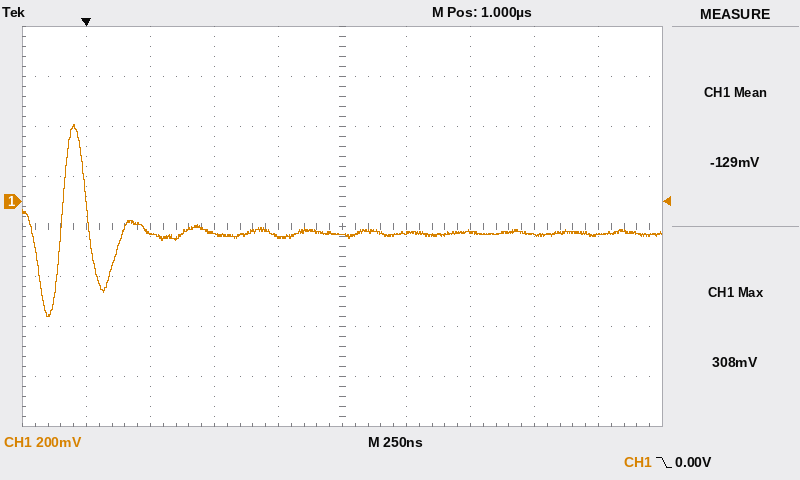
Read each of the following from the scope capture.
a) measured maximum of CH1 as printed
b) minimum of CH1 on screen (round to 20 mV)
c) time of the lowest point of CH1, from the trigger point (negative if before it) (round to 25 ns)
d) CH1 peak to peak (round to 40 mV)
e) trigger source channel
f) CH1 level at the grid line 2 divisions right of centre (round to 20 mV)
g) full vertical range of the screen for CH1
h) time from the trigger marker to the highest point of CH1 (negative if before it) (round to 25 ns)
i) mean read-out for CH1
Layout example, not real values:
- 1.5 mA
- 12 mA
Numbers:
- 308 mV
- -460 mV
- -150 ns
- 760 mV
- CH1
- -120 mV
- 1.6 V
- -50 ns
- -129 mV
